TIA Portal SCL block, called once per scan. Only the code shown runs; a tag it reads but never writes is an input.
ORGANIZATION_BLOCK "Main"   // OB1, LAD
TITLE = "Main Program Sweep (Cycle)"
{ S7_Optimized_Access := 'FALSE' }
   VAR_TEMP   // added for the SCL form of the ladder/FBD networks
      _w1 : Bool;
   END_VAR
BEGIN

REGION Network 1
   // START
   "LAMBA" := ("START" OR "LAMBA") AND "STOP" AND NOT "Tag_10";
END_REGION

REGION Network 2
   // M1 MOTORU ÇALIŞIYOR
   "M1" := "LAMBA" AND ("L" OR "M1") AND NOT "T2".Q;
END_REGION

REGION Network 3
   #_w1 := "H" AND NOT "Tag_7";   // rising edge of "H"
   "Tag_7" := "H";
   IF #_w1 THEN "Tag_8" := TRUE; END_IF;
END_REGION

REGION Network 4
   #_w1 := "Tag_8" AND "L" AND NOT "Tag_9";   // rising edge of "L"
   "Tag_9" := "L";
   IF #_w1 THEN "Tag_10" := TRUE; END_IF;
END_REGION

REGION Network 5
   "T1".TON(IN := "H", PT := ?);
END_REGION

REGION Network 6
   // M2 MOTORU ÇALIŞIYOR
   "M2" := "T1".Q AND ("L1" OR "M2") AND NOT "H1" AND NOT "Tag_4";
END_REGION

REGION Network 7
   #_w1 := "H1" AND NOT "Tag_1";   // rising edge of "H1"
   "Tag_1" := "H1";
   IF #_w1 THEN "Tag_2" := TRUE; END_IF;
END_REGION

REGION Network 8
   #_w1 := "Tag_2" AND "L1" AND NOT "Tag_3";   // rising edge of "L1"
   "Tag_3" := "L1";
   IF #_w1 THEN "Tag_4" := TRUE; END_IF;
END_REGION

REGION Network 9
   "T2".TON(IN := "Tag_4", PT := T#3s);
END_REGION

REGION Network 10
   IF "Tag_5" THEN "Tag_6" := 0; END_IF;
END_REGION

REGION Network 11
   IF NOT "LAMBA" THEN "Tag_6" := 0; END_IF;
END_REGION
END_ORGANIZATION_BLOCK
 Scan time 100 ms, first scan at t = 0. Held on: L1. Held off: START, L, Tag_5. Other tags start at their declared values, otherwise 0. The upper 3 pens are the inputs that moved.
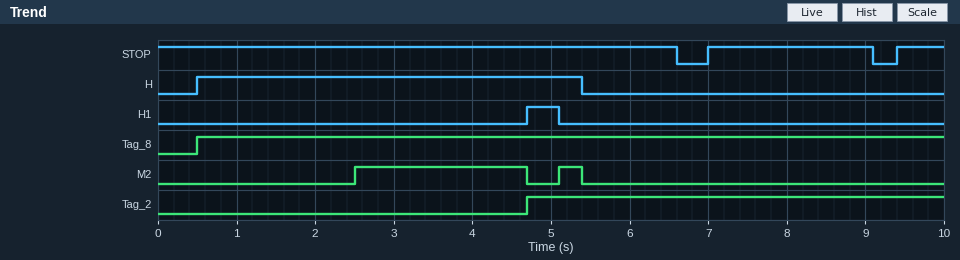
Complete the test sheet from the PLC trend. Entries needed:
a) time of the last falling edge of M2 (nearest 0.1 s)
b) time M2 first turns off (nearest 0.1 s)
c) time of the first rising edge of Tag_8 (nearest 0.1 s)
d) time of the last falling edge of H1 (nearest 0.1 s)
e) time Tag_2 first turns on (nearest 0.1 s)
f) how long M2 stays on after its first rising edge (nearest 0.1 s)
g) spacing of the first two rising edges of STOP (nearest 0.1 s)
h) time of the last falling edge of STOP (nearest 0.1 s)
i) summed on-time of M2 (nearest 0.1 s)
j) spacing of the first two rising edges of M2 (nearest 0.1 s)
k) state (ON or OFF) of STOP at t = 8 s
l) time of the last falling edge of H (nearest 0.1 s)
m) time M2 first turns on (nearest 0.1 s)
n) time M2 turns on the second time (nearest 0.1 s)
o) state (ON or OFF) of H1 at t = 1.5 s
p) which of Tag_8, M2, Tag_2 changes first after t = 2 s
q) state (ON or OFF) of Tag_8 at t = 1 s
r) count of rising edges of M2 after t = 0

5.4 s
4.7 s
0.5 s
5.1 s
4.7 s
2.2 s
2.4 s
9.1 s
2.5 s
2.6 s
ON
5.4 s
2.5 s
5.1 s
OFF
M2
ON
2
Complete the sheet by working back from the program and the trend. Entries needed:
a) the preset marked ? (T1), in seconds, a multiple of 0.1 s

2.0 s
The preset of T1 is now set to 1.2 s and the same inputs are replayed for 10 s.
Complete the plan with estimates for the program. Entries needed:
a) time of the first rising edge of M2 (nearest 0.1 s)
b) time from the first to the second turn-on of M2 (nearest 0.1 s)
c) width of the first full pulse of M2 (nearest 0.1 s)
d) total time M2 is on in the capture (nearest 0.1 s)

1.7 s
3.4 s
3.0 s
3.3 s
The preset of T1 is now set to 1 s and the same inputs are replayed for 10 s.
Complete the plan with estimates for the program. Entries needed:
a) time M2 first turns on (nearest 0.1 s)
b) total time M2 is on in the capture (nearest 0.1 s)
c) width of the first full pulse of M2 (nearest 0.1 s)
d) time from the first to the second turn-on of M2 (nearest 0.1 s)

1.5 s
3.5 s
3.2 s
3.6 s
